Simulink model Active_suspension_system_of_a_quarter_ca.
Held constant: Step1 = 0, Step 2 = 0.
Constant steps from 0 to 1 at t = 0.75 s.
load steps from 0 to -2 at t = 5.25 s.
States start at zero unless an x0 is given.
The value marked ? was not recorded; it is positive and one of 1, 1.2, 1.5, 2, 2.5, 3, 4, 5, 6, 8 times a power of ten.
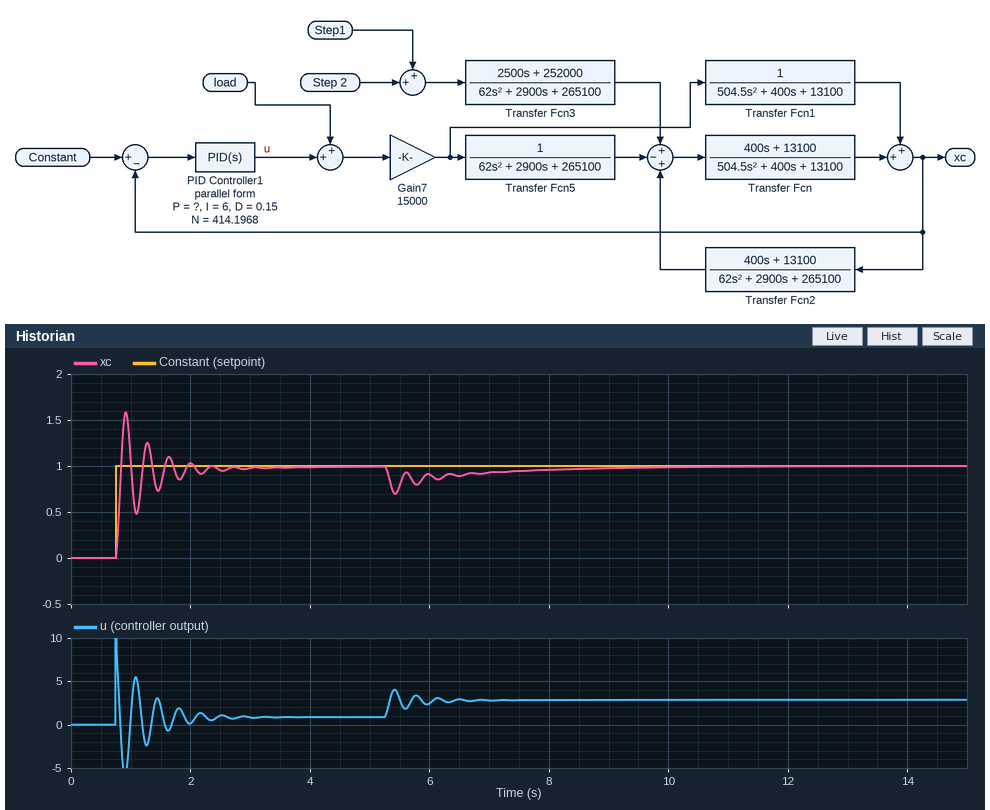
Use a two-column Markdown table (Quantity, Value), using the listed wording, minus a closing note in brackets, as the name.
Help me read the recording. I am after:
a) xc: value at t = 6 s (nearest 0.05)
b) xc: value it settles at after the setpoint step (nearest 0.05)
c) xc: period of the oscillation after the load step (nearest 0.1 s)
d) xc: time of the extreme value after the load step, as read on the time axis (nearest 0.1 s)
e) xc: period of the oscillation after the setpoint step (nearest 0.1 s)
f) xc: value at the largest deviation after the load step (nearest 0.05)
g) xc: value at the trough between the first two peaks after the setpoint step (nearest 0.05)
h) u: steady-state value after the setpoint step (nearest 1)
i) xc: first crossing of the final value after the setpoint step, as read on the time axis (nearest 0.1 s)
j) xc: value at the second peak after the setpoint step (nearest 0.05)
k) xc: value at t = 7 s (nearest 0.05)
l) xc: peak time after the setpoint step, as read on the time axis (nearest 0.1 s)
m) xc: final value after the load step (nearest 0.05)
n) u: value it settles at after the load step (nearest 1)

| Quantity | Value |
|---|---|
| xc: value at t = 6 s | 0.90 |
| xc: value it settles at after the setpoint step | 1.00 |
| xc: period of the oscillation after the load step | 0.4 s |
| xc: time of the extreme value after the load step, as read on the time axis | 5.4 s |
| xc: period of the oscillation after the setpoint step | 0.4 s |
| xc: value at the largest deviation after the load step | 0.70 |
| xc: value at the trough between the first two peaks after the setpoint step | 0.50 |
| u: steady-state value after the setpoint step | 1 |
| xc: first crossing of the final value after the setpoint step, as read on the time axis | 0.8 s |
| xc: value at the second peak after the setpoint step | 1.25 |
| xc: value at t = 7 s | 0.95 |
| xc: peak time after the setpoint step, as read on the time axis | 0.9 s |
| xc: final value after the load step | 1.00 |
| u: value it settles at after the load step | 3 |
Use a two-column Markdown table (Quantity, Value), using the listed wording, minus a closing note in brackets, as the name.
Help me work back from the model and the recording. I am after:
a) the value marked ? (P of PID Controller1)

| Quantity | Value |
|---|---|
| the value marked ? | 10 |
